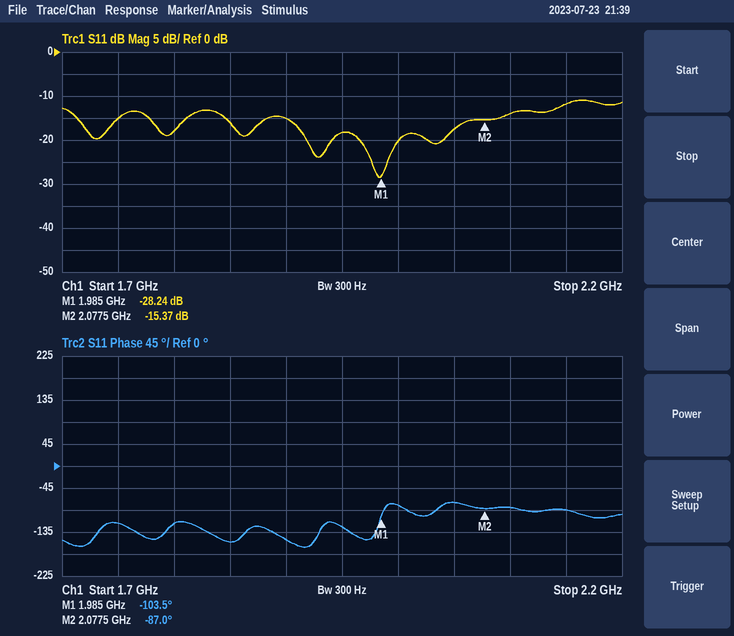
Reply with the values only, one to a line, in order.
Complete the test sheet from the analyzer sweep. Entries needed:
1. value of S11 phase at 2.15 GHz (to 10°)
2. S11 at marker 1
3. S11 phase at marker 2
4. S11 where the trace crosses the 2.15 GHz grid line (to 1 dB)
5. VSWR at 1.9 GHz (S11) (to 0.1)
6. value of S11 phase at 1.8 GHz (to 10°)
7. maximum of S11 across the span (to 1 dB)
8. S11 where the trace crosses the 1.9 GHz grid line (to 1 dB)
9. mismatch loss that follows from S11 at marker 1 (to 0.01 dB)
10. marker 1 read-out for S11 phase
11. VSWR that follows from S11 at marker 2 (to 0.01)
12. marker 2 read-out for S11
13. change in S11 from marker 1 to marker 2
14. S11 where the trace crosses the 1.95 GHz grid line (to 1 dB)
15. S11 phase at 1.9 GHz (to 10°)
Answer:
-90°
-28.24 dB
-87.0°
-12 dB
1.4
-120°
-11 dB
-15 dB
0.01 dB
-103.5°
1.41
-15.37 dB
12.87 dB
-18 dB
-150°
